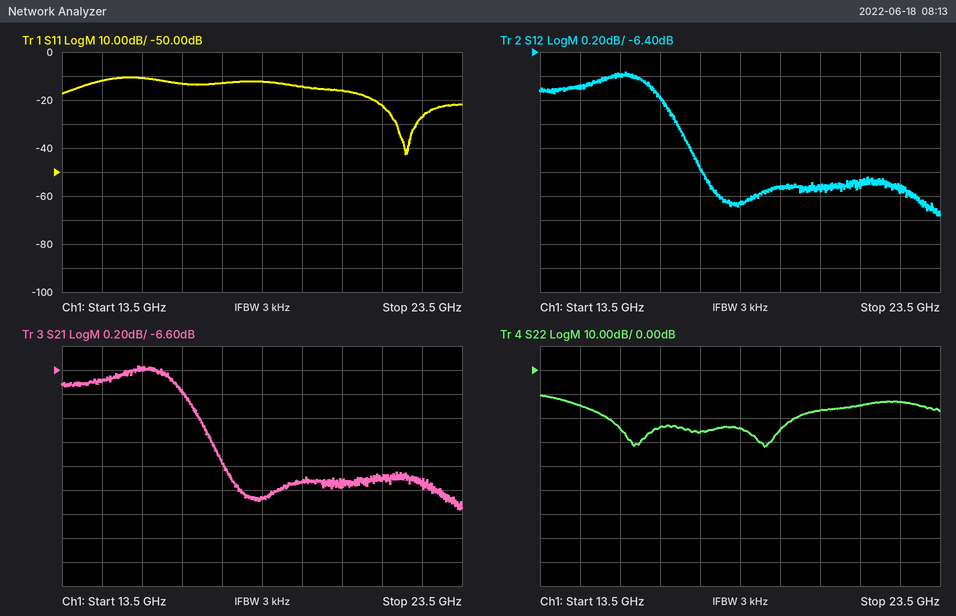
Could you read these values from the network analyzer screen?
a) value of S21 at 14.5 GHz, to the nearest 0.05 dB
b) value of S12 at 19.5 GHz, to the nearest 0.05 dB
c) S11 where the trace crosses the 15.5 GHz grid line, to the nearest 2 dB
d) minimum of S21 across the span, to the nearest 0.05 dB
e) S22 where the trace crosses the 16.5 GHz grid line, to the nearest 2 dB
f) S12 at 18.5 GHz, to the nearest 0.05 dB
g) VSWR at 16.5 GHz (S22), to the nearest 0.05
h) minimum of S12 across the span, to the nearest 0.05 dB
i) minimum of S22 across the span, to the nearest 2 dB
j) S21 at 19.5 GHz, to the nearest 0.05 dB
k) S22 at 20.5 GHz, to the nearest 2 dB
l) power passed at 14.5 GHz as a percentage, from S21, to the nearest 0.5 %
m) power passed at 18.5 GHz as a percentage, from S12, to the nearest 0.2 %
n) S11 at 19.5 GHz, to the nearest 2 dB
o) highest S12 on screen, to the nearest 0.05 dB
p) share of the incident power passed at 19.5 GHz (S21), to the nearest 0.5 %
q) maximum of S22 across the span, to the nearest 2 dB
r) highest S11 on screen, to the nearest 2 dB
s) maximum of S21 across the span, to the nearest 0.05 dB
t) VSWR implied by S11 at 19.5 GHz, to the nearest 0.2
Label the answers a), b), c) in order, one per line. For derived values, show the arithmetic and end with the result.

a) -6.70 dB
b) -7.55 dB
c) -10 dB
d) -7.75 dB
e) -24 dB
f) -7.65 dB
g) |Γ| = 10^(-24/20) = 0.0631; VSWR = (1 + 0.0631)/(1 − 0.0631) ≈ 1.13, so 1.15 to the nearest 0.05
h) -7.75 dB
i) -32 dB
j) -7.55 dB
k) -16 dB
l) 10^(-6.7/10) ≈ 21.4 %, so 21.5 % to the nearest 0.5 %
m) 10^(-7.65/10) ≈ 17.2 %
n) -14 dB
o) -6.55 dB
p) 10^(-7.55/10) ≈ 17.6 %, so 17.5 % to the nearest 0.5 %
q) -10 dB
r) -10 dB
s) -6.55 dB
t) |Γ| = 10^(-14/20) = 0.1995; VSWR = (1 + 0.1995)/(1 − 0.1995) ≈ 1.50, so 1.4 to the nearest 0.2
